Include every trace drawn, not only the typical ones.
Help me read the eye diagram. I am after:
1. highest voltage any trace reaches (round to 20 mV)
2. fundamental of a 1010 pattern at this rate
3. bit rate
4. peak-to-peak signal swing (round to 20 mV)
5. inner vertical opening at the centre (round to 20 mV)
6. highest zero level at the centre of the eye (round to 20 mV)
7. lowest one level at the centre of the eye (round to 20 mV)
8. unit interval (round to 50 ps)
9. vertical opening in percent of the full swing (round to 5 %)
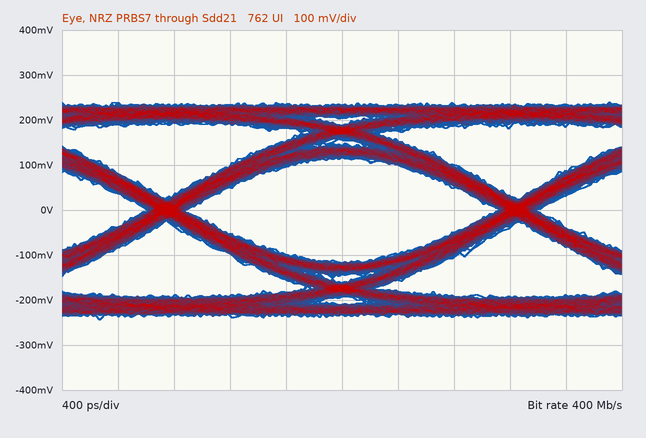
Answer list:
240 mV
200 MHz
400 Mb/s
480 mV
240 mV
-120 mV
120 mV
2.50 ns
50 %
